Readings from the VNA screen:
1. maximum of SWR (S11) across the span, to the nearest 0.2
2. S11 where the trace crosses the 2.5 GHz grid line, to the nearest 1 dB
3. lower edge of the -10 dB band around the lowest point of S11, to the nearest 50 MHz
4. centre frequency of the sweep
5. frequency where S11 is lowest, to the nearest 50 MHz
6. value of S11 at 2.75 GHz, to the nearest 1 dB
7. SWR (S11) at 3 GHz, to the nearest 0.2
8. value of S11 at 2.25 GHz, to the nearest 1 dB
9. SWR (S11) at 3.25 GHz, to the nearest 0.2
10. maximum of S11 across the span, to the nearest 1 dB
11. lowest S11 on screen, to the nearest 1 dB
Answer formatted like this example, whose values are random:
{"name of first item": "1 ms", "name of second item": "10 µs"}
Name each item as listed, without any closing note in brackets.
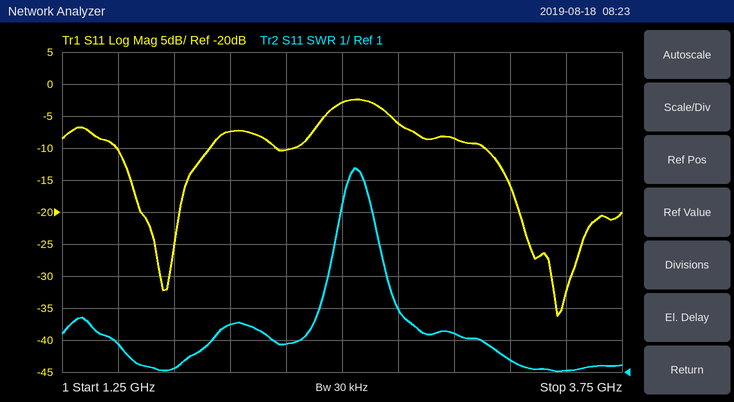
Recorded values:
{"maximum of SWR (S11) across the span, to the nearest 0.2": "7.4", "S11 where the trace crosses the 2.5 GHz grid line, to the nearest 1 dB": "-3 dB", "lower edge of the -10 dB band around the lowest point of S11, to the nearest 50 MHz": "3.15 GHz", "centre frequency of the sweep": "2.5 GHz", "frequency where S11 is lowest, to the nearest 50 MHz": "3.45 GHz", "value of S11 at 2.75 GHz, to the nearest 1 dB": "-6 dB", "SWR (S11) at 3 GHz, to the nearest 0.2": "2.2", "value of S11 at 2.25 GHz, to the nearest 1 dB": "-10 dB", "SWR (S11) at 3.25 GHz, to the nearest 0.2": "1.4", "maximum of S11 across the span, to the nearest 1 dB": "-2 dB", "lowest S11 on screen, to the nearest 1 dB": "-36 dB"}
